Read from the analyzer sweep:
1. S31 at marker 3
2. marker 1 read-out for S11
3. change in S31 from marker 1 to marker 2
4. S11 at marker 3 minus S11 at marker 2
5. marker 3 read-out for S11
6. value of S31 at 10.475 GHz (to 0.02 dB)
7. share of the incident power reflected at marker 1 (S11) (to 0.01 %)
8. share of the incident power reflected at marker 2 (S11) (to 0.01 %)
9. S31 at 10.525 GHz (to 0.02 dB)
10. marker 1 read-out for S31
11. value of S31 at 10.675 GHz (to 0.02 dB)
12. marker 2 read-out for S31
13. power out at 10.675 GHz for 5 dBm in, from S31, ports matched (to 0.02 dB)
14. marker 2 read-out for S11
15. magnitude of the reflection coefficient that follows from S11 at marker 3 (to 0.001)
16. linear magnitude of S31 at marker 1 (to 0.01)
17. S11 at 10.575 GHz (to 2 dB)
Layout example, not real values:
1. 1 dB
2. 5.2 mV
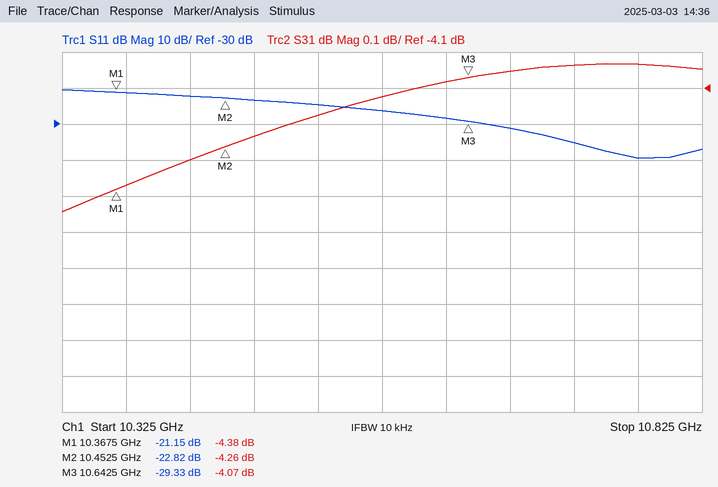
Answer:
1. -4.07 dB
2. -21.15 dB
3. 0.12 dB
4. -6.51 dB
5. -29.33 dB
6. -4.24 dB
7. 0.77 %
8. 0.52 %
9. -4.18 dB
10. -4.38 dB
11. -4.06 dB
12. -4.26 dB
13. 0.94 dBm
14. -22.82 dB
15. 0.034
16. 0.60
17. -26 dB
